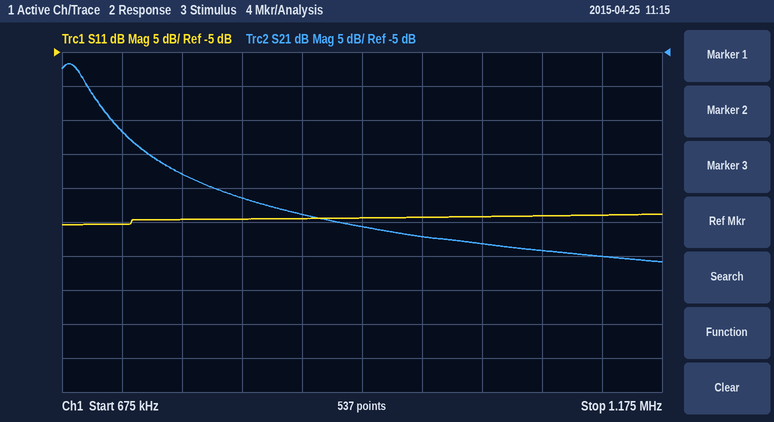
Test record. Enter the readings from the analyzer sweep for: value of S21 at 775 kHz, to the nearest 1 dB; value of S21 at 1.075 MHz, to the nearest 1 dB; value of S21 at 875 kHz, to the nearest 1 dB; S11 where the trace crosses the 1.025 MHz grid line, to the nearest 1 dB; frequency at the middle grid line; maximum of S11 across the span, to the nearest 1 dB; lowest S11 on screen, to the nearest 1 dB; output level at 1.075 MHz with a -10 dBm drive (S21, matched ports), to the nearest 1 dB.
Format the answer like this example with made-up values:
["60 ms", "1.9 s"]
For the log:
["-23 dB", "-34 dB", "-29 dB", "-29 dB", "925 kHz", "-29 dB", "-30 dB", "-44 dBm"]
